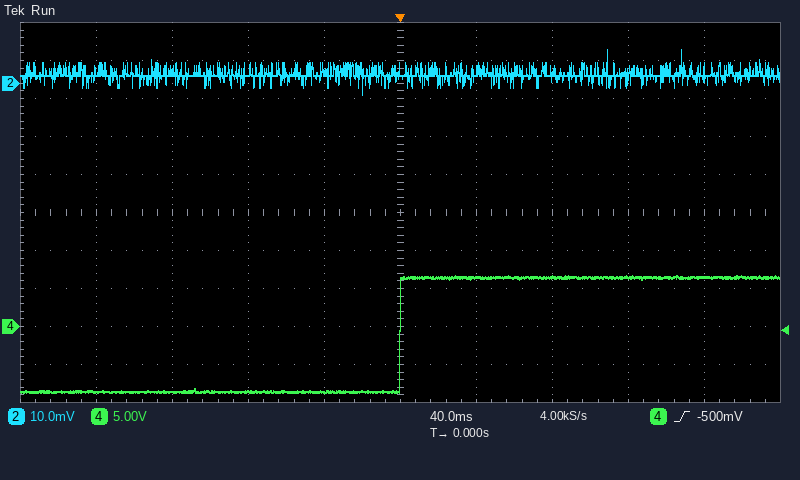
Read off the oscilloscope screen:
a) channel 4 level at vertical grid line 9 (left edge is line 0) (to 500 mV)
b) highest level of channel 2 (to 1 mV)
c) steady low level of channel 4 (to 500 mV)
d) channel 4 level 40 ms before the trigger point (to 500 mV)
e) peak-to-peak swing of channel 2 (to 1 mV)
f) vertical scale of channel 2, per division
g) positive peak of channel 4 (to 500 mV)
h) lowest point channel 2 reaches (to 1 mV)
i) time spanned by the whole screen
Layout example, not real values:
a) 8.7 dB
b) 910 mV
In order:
a) 6.5 V
b) 9 mV
c) -8.5 V
d) -8.5 V
e) 12 mV
f) 10 mV
g) 6.5 V
h) -3 mV
i) 400 ms
